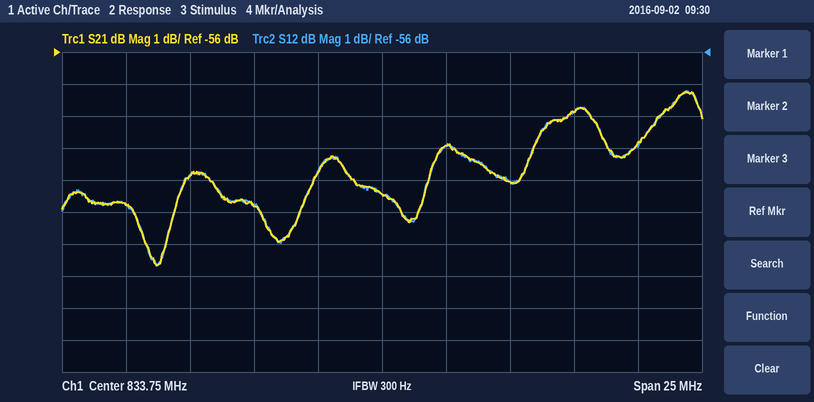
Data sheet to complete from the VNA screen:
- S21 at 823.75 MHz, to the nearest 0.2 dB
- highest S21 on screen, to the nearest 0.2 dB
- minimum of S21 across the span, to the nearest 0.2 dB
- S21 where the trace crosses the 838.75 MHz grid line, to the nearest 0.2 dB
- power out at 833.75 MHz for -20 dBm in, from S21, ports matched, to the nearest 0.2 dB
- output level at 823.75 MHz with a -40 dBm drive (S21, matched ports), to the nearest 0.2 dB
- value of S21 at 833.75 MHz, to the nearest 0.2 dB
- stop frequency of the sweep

-60.8 dB
-57.2 dB
-62.6 dB
-60.0 dB
-80.4 dBm
-100.8 dBm
-60.4 dB
846.25 MHz
